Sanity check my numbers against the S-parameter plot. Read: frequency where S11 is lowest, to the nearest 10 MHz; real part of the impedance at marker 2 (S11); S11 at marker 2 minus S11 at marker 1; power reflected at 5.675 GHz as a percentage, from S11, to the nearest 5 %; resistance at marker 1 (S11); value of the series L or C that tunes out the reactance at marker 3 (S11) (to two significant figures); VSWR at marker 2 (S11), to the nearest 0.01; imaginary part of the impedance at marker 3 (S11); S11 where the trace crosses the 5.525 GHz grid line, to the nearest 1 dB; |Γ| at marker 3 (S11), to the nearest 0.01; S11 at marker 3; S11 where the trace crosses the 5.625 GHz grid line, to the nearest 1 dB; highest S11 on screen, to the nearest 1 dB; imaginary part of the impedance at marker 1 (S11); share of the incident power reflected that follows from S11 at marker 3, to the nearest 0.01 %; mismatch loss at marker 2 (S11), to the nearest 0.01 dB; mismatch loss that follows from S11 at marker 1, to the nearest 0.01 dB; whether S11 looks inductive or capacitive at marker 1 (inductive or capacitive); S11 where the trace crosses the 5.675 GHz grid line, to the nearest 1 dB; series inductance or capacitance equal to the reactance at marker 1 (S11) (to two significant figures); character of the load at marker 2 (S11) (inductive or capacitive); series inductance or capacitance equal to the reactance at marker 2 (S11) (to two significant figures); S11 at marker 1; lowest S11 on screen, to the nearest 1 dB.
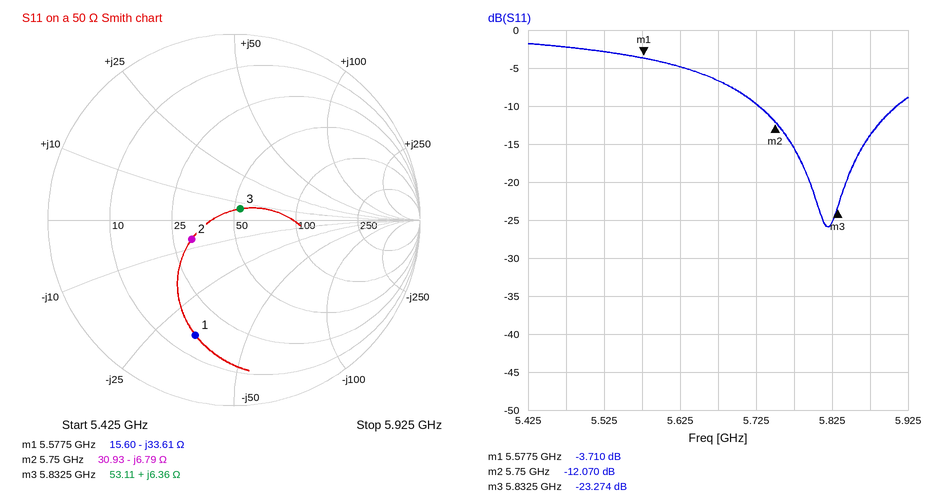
5.82 GHz
30.93 Ω
-8.360 dB
20 %
15.60 Ω
4.3 pF
1.66
+6.36 Ω
-3 dB
0.07
-23.274 dB
-5 dB
-2 dB
-33.61 Ω
0.47 %
0.28 dB
2.41 dB
capacitive
-7 dB
850 fF
capacitive
4.1 pF
-3.710 dB
-26 dB
